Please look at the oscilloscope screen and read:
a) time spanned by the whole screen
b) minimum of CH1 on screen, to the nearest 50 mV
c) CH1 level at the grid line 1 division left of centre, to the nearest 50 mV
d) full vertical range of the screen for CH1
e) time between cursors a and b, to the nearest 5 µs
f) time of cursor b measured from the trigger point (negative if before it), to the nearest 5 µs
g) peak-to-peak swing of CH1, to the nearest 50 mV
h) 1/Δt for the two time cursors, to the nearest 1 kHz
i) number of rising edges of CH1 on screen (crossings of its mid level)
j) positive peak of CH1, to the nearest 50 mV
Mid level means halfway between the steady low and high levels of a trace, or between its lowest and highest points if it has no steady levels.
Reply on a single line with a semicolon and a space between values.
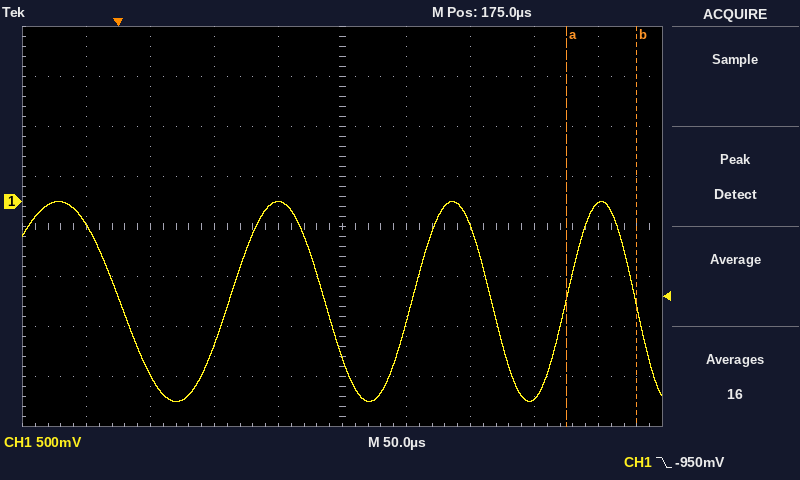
500 µs; -2.00 V; 0 mV; 4 V; 55 µs; +405 µs; 2.00 V; 18 kHz; 3; 0 mV
